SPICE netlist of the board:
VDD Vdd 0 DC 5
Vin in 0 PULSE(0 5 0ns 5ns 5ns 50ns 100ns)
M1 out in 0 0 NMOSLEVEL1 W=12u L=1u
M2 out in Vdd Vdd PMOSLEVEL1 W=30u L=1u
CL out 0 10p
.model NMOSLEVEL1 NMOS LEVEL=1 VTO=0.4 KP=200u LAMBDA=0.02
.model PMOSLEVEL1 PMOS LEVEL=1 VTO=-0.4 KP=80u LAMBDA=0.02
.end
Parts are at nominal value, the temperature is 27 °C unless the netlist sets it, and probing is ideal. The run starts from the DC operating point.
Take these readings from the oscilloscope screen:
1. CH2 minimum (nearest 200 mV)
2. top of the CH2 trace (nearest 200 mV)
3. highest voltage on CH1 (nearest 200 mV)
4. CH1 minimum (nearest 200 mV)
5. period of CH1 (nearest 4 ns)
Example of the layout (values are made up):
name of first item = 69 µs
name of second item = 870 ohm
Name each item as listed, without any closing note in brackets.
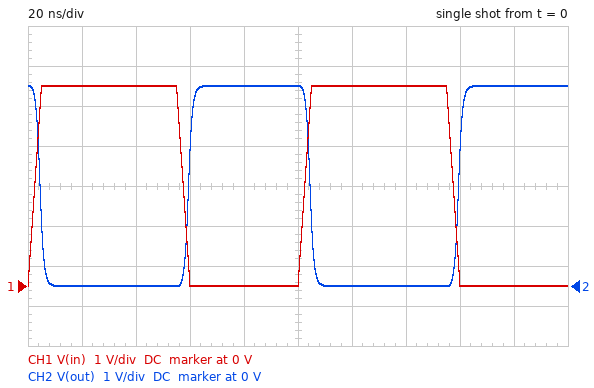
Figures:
CH2 minimum = 0 V
top of the CH2 trace = 5.0 V
highest voltage on CH1 = 5.0 V
CH1 minimum = 0 V
period of CH1 = 100 ns
